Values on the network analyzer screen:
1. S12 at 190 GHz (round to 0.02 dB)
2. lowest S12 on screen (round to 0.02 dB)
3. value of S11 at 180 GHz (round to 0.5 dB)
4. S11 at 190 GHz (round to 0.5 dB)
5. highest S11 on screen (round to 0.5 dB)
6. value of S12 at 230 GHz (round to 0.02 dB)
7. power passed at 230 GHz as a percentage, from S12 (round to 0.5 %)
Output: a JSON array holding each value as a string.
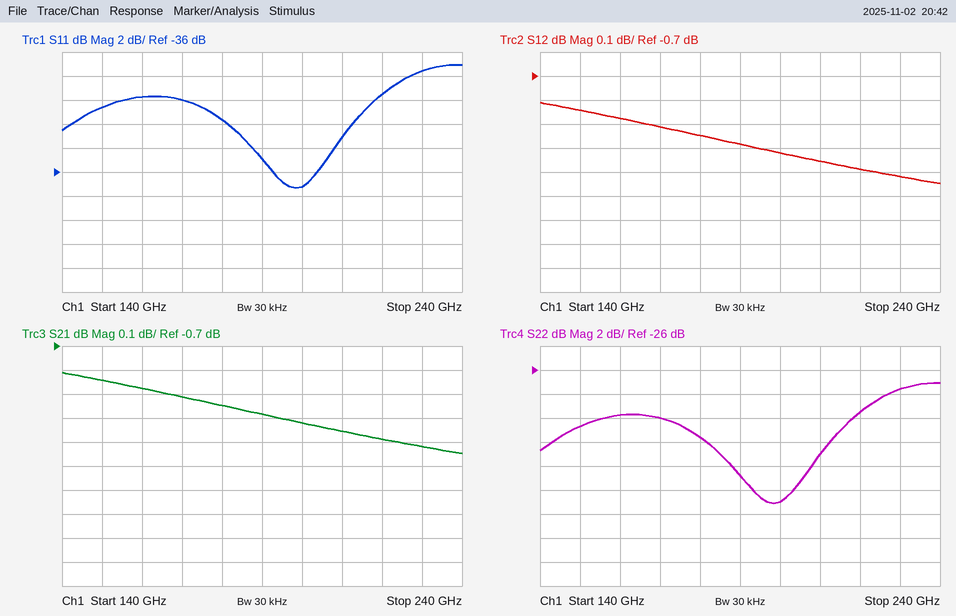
["-0.98 dB", "-1.14 dB", "-31.5 dB", "-35.0 dB", "-27.0 dB", "-1.12 dB", "77.5 %"]
